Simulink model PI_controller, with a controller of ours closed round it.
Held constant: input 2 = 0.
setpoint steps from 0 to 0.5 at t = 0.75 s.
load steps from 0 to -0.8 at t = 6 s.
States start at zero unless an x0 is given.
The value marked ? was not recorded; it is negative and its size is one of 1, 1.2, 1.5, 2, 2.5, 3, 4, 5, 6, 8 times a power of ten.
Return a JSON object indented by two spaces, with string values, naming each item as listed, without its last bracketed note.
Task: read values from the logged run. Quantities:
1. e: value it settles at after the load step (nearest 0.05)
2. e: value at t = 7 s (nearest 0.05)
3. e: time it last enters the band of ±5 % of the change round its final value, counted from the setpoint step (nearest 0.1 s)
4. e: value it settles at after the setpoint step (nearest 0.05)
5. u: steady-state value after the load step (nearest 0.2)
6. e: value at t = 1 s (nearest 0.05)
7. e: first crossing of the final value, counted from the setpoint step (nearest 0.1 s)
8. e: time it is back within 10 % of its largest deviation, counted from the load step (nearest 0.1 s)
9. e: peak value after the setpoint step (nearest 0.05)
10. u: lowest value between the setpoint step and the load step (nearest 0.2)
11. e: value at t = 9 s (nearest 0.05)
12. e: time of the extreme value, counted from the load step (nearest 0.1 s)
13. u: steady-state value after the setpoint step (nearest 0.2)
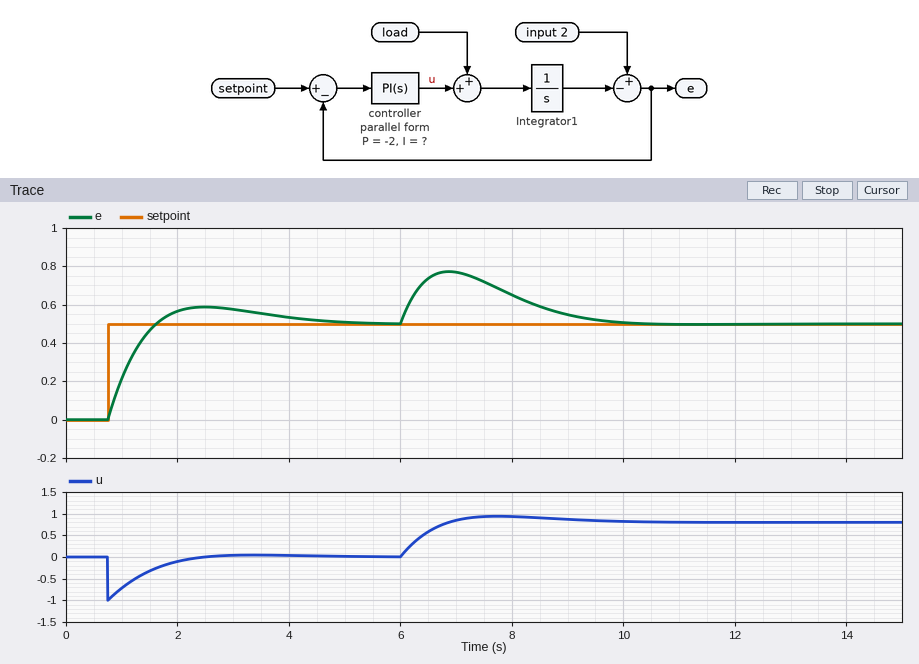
{
  "e: value it settles at after the load step": "0.50",
  "e: value at t = 7 s": "0.75",
  "e: time it last enters the band of ±5 % of the change round its final value, counted from the setpoint step": "3.5 s",
  "e: value it settles at after the setpoint step": "0.50",
  "u: steady-state value after the load step": "0.8",
  "e: value at t = 1 s": "0.20",
  "e: first crossing of the final value, counted from the setpoint step": "0.9 s",
  "e: time it is back within 10 % of its largest deviation, counted from the load step": "3.4 s",
  "e: peak value after the setpoint step": "0.60",
  "u: lowest value between the setpoint step and the load step": "-1.0",
  "e: value at t = 9 s": "0.55",
  "e: time of the extreme value, counted from the load step": "0.9 s",
  "u: steady-state value after the setpoint step": "0.0"
}
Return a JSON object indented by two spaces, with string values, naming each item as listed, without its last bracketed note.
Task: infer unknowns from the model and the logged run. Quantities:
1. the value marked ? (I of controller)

{
  "the value marked ?": "-1.5"
}
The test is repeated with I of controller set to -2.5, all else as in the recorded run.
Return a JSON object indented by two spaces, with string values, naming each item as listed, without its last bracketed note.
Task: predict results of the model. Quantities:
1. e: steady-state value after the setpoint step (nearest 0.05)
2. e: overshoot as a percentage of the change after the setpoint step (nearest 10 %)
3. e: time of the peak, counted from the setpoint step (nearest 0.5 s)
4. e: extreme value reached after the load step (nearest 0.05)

{
  "e: steady-state value after the setpoint step": "0.50",
  "e: overshoot as a percentage of the change after the setpoint step": "20 %",
  "e: time of the peak, counted from the setpoint step": "1.5 s",
  "e: extreme value reached after the load step": "0.75"
}
